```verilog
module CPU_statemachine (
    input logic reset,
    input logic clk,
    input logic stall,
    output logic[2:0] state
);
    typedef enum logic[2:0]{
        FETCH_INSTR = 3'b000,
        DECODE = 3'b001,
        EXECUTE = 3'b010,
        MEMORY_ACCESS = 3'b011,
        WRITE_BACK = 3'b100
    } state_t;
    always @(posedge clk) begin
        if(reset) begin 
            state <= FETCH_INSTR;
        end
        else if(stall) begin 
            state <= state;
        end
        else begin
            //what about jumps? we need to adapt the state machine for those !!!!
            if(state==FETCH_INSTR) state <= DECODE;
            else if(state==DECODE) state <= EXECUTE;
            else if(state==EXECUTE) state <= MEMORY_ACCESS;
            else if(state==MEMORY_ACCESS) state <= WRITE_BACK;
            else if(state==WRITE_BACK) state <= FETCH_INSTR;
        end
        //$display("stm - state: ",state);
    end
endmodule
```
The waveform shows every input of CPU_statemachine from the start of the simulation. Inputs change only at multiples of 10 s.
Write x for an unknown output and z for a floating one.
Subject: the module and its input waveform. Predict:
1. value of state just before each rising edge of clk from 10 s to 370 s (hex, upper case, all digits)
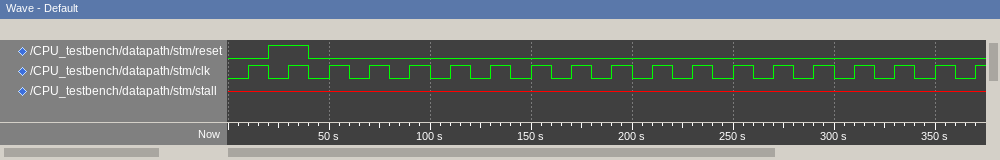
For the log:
x, x, 0, 1, 2, 3, 4, 0, 1, 2, 3, 4, 0, 1, 2, 3, 4, 0, 1
